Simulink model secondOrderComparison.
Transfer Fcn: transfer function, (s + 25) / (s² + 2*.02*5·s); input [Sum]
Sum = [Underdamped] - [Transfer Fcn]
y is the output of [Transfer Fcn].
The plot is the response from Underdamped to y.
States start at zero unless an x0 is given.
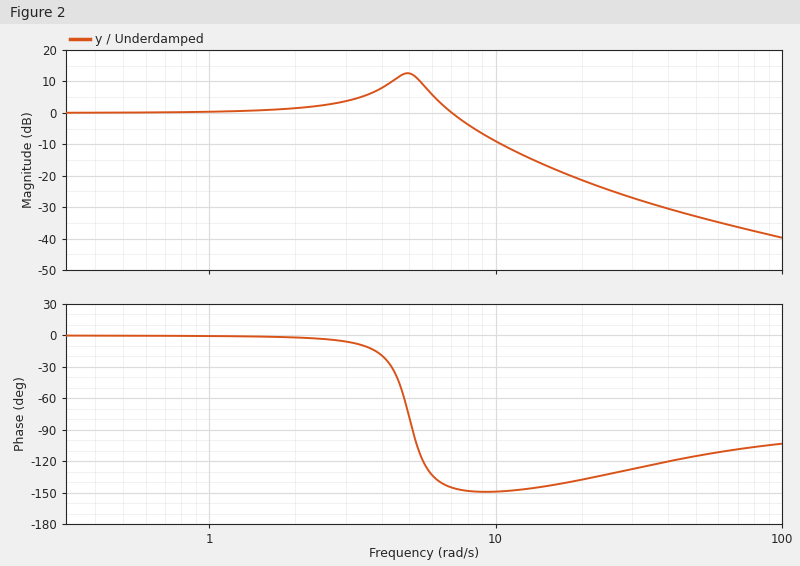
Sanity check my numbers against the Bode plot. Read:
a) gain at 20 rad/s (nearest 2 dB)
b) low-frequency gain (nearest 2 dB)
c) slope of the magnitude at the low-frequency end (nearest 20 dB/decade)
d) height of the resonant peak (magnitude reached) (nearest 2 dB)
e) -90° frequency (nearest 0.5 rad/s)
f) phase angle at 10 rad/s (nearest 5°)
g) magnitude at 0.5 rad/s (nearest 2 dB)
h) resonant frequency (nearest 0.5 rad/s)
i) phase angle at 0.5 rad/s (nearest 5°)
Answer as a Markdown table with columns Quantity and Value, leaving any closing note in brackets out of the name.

| Quantity | Value |
|---|---|
| gain at 20 rad/s | -22 dB |
| low-frequency gain | 0 dB |
| slope of the magnitude at the low-frequency end | 0 dB/decade |
| height of the resonant peak (magnitude reached) | 12 dB |
| -90° frequency | 5.0 rad/s |
| phase angle at 10 rad/s | -150° |
| magnitude at 0.5 rad/s | 0 dB |
| resonant frequency | 5.0 rad/s |
| phase angle at 0.5 rad/s | 0° |
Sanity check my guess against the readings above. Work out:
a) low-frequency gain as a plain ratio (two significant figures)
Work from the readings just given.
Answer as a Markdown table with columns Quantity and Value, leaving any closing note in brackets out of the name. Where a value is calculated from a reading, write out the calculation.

| Quantity | Value |
|---|---|
| low-frequency gain as a plain ratio | 10^(0 / 20) = 1.0 |
